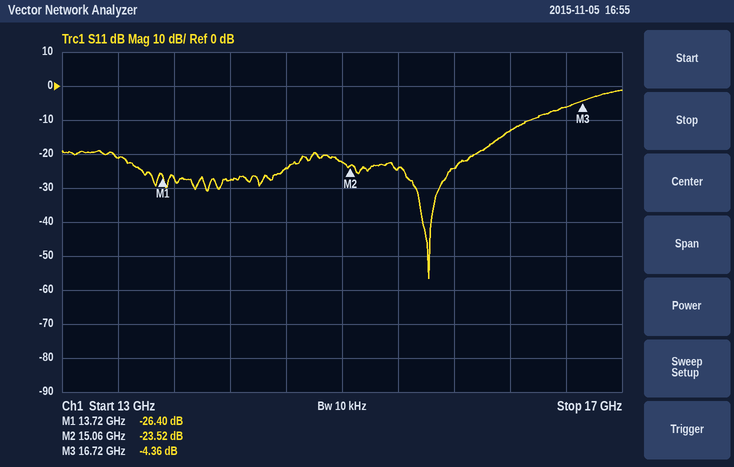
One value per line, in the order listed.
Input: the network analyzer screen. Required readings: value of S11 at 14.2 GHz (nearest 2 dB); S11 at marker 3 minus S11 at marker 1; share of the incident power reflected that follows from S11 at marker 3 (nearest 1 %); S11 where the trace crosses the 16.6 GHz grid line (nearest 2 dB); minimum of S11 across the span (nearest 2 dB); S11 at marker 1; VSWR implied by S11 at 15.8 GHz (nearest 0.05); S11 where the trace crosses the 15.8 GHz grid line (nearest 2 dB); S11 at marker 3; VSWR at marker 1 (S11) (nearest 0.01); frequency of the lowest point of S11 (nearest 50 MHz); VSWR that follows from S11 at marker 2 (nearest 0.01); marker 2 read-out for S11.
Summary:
-28 dB
22.04 dB
37 %
-6 dB
-56 dB
-26.40 dB
1.15
-24 dB
-4.36 dB
1.10
15.60 GHz
1.14
-23.52 dB
